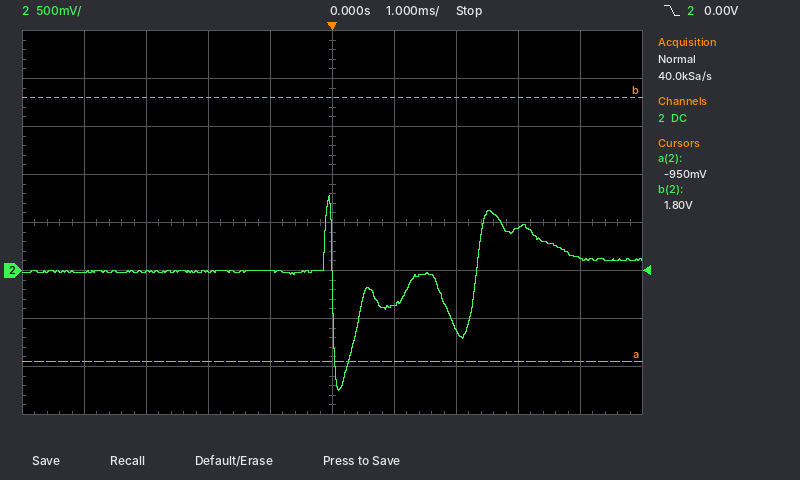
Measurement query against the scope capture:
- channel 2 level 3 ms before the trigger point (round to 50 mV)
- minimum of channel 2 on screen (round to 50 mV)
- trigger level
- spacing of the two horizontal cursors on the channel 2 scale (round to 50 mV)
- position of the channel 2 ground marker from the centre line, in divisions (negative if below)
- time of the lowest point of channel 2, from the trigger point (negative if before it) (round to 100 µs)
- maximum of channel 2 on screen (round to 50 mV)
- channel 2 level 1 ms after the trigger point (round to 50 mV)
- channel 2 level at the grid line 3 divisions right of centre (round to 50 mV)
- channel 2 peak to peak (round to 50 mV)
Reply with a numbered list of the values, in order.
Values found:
1. 0 mV
2. -1.25 V
3. 0.00 V
4. 2.75 V
5. -1.0 div
6. +100 µs
7. 800 mV
8. -350 mV
9. 450 mV
10. 2.05 V
